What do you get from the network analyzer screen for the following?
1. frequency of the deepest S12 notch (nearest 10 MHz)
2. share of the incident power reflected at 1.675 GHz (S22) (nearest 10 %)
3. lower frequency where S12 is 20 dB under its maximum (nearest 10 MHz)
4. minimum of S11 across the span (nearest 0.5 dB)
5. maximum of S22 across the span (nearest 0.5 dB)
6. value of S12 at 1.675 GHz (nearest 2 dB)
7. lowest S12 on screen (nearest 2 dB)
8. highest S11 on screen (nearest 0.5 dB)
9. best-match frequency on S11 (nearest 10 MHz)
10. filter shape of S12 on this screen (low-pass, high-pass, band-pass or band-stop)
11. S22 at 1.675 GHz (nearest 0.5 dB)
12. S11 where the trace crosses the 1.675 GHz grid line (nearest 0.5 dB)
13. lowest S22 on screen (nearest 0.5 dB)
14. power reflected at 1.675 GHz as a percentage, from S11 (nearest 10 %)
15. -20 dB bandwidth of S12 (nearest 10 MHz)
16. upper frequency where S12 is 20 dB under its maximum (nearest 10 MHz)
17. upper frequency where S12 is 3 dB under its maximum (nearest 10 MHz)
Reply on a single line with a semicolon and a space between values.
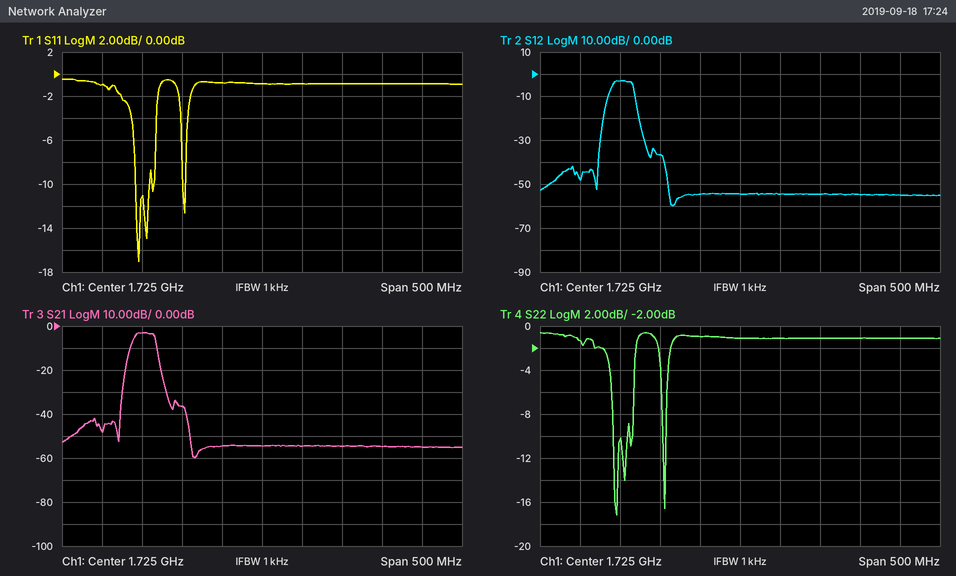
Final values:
1.64 GHz; 80 %; 1.55 GHz; -17.0 dB; -0.5 dB; -54 dB; -60 dB; -0.5 dB; 1.57 GHz; band-pass; -1.0 dB; -1.0 dB; -17.0 dB; 80 %; 50 MHz; 1.60 GHz; 1.59 GHz
